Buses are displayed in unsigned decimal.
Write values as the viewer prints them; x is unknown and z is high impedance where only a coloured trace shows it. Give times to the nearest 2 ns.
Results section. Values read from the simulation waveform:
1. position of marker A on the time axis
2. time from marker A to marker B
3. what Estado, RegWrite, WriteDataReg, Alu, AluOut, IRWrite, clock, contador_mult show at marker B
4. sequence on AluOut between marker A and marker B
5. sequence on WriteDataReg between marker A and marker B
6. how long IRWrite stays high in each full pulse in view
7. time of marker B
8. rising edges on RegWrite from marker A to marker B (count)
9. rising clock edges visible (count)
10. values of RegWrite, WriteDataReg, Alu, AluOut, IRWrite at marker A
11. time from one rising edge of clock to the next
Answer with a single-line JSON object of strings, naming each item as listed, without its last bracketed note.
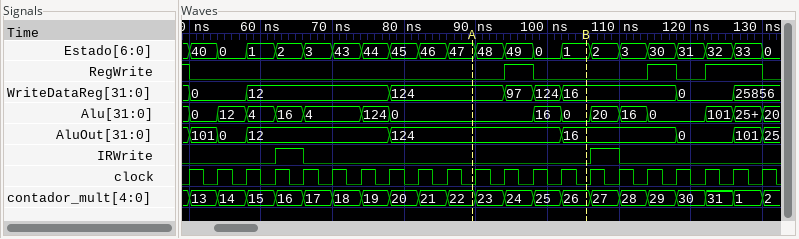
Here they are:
{"position of marker A on the time axis": "90 ns", "time from marker A to marker B": "16 ns", "what Estado, RegWrite, WriteDataReg, Alu, AluOut, IRWrite, clock, contador_mult show at marker B": "Estado=1, RegWrite=0, WriteDataReg=16, Alu=0, AluOut=16, IRWrite=0, clock=0, contador_mult=26", "sequence on AluOut between marker A and marker B": "124, 16", "sequence on WriteDataReg between marker A and marker B": "124, 97, 124, 16", "how long IRWrite stays high in each full pulse in view": "4 ns, 4 ns", "time of marker B": "106 ns", "rising edges on RegWrite from marker A to marker B": "1", "rising clock edges visible": "21", "values of RegWrite, WriteDataReg, Alu, AluOut, IRWrite at marker A": "RegWrite=0, WriteDataReg=124, Alu=0, AluOut=124, IRWrite=0", "time from one rising edge of clock to the next": "4 ns"}
